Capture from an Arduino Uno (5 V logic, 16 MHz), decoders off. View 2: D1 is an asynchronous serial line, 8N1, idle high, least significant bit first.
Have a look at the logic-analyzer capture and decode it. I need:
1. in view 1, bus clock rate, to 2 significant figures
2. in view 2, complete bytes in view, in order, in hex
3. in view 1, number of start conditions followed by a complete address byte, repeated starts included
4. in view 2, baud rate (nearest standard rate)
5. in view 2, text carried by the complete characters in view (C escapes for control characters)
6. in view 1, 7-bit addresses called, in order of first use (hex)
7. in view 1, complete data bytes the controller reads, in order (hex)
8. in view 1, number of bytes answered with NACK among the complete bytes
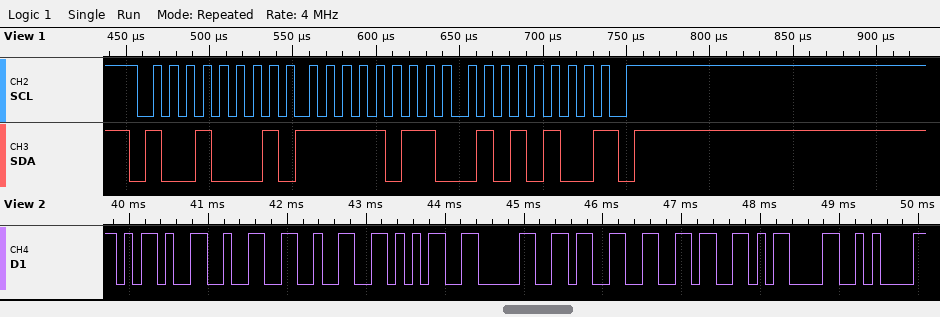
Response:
100 kHz
2D 32 32 35 30 33 36 0D 0A
1
9600 baud
"-225036\r\n"
0x48
FB 54
1
